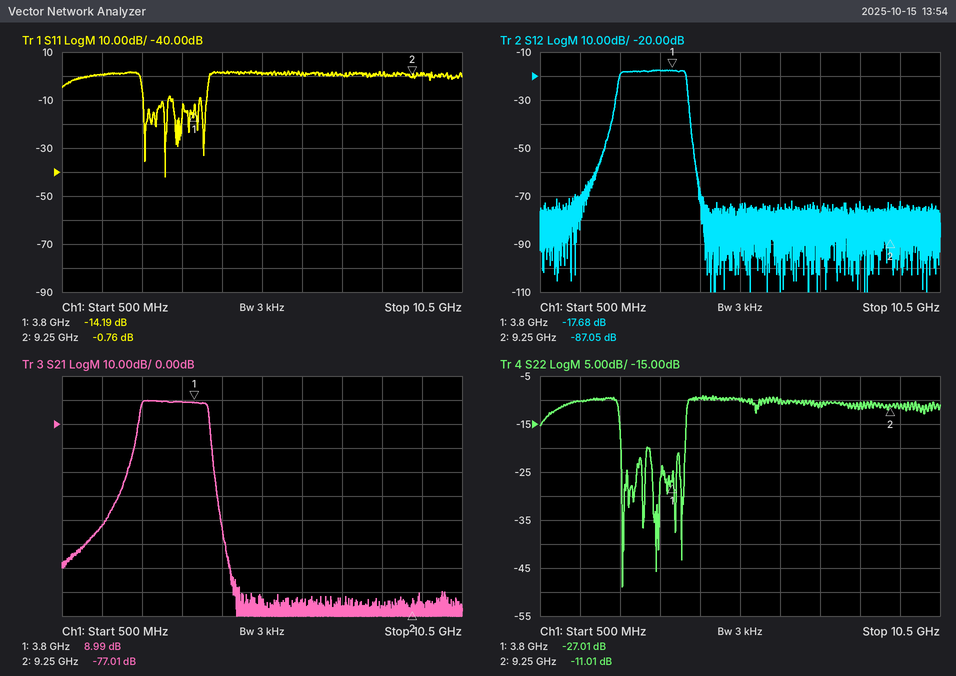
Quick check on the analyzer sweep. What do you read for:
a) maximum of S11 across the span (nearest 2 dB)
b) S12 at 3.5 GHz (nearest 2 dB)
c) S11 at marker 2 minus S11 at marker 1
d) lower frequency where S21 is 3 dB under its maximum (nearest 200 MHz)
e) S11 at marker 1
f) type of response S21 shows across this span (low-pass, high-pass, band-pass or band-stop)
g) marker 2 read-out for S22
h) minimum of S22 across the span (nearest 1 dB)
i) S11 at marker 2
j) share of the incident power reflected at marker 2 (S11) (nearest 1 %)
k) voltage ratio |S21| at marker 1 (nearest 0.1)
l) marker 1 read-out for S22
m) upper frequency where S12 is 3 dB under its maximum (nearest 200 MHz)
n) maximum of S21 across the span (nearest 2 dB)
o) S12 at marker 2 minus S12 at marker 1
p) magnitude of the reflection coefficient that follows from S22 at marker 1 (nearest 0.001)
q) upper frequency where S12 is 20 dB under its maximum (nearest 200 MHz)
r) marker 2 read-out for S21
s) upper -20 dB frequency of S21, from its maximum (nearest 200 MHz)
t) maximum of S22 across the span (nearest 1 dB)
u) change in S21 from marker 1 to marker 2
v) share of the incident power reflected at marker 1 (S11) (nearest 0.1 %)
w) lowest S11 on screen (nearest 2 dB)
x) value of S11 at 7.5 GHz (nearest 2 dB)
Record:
2 dB
-18 dB
13.43 dB
2.4 GHz
-14.19 dB
band-pass
-11.01 dB
-49 dB
-0.76 dB
84 %
2.8
-27.01 dB
4.2 GHz
10 dB
-69.37 dB
0.045
4.2 GHz
-77.01 dB
4.2 GHz
-9 dB
-86.00 dB
3.8 %
-42 dB
0 dB
